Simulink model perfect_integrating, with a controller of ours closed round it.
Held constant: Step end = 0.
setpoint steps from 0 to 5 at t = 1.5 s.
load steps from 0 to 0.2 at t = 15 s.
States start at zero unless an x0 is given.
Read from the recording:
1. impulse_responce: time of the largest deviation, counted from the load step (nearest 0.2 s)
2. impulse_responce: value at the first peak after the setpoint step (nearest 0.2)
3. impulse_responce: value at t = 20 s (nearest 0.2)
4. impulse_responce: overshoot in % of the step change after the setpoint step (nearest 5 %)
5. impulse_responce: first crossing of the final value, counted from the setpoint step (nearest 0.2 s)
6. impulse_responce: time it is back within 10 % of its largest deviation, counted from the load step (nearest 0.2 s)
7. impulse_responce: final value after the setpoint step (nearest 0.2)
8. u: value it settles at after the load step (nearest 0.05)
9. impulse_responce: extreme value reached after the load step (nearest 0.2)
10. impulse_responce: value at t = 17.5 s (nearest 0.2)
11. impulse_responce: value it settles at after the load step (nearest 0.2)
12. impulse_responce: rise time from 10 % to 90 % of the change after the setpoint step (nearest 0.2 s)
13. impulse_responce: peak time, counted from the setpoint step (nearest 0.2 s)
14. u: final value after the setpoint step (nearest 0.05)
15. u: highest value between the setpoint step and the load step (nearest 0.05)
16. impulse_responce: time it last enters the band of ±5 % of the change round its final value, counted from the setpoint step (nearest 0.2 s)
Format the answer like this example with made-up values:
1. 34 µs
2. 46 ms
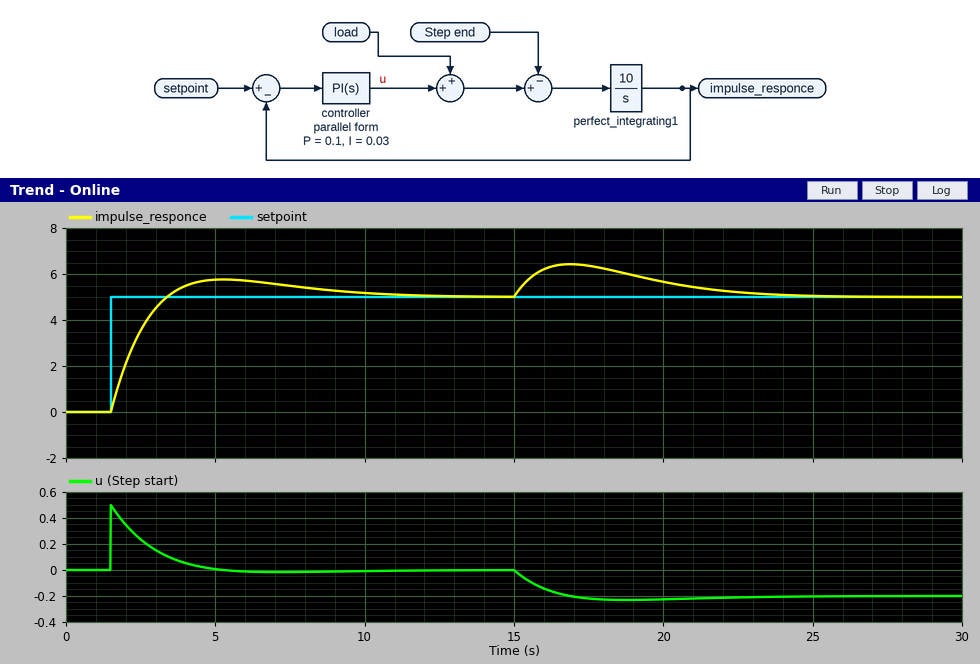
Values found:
1. 1.8 s
2. 5.8
3. 5.6
4. 15 %
5. 1.8 s
6. 8.2 s
7. 5.0
8. -0.20
9. 6.4
10. 6.4
11. 5.0
12. 1.4 s
13. 3.8 s
14. 0.00
15. 0.50
16. 7.8 s
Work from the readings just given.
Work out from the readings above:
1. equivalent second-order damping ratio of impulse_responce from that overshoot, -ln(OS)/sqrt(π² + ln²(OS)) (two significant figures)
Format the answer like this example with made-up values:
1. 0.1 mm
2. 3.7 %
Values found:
1. 0.52
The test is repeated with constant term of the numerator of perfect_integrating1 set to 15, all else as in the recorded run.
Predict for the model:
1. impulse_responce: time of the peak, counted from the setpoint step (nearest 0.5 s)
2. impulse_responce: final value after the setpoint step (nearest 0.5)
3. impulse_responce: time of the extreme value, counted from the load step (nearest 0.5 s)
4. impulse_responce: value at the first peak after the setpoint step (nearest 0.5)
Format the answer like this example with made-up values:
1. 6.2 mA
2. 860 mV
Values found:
1. 3.0 s
2. 5.0
3. 1.5 s
4. 5.5
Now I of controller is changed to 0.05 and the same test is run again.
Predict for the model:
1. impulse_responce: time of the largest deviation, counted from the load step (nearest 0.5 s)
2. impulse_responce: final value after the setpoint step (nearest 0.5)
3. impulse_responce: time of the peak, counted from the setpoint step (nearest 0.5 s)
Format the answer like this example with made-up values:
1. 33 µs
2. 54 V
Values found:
1. 1.5 s
2. 5.0
3. 3.0 s
